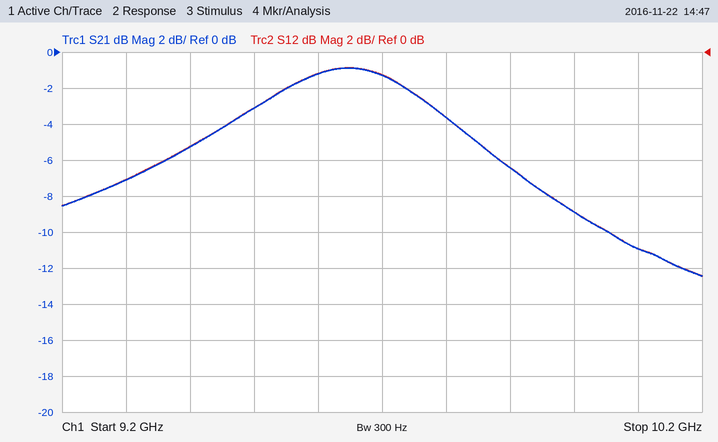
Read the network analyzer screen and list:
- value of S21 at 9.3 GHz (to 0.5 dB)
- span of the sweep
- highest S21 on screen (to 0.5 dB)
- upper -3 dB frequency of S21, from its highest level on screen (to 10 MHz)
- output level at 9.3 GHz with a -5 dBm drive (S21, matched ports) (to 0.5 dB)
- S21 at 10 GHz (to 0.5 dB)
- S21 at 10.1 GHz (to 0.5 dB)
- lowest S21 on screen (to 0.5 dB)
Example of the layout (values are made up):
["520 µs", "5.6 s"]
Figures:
["-7.0 dB", "1 GHz", "-1.0 dB", "9.81 GHz", "-12.0 dBm", "-9.0 dB", "-11.0 dB", "-12.5 dB"]
